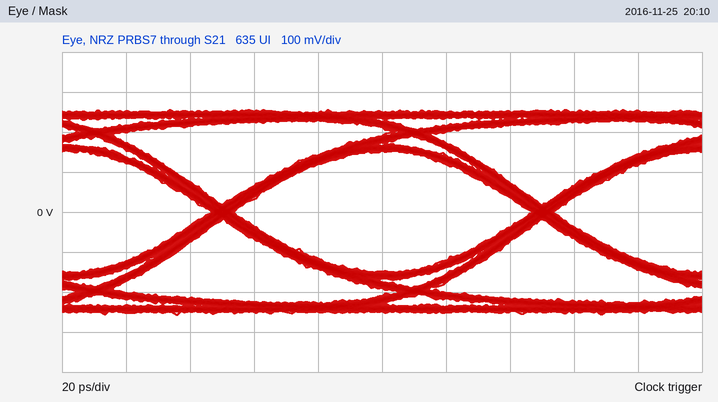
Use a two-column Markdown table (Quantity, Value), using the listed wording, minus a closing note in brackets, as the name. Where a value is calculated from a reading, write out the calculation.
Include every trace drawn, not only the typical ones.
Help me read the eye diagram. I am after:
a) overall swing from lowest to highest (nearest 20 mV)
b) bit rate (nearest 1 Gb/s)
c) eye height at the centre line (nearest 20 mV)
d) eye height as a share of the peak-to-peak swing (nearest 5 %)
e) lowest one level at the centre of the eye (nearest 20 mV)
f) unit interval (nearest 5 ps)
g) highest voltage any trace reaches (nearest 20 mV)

| Quantity | Value |
|---|---|
| overall swing from lowest to highest | 520 mV |
| bit rate | 10 Gb/s |
| eye height at the centre line | 300 mV |
| eye height as a share of the peak-to-peak swing | 300 mV / 520 mV ≈ 57.7 %, so 60 % to the nearest 5 % |
| lowest one level at the centre of the eye | 160 mV |
| unit interval | 100 ps |
| highest voltage any trace reaches | 260 mV |
